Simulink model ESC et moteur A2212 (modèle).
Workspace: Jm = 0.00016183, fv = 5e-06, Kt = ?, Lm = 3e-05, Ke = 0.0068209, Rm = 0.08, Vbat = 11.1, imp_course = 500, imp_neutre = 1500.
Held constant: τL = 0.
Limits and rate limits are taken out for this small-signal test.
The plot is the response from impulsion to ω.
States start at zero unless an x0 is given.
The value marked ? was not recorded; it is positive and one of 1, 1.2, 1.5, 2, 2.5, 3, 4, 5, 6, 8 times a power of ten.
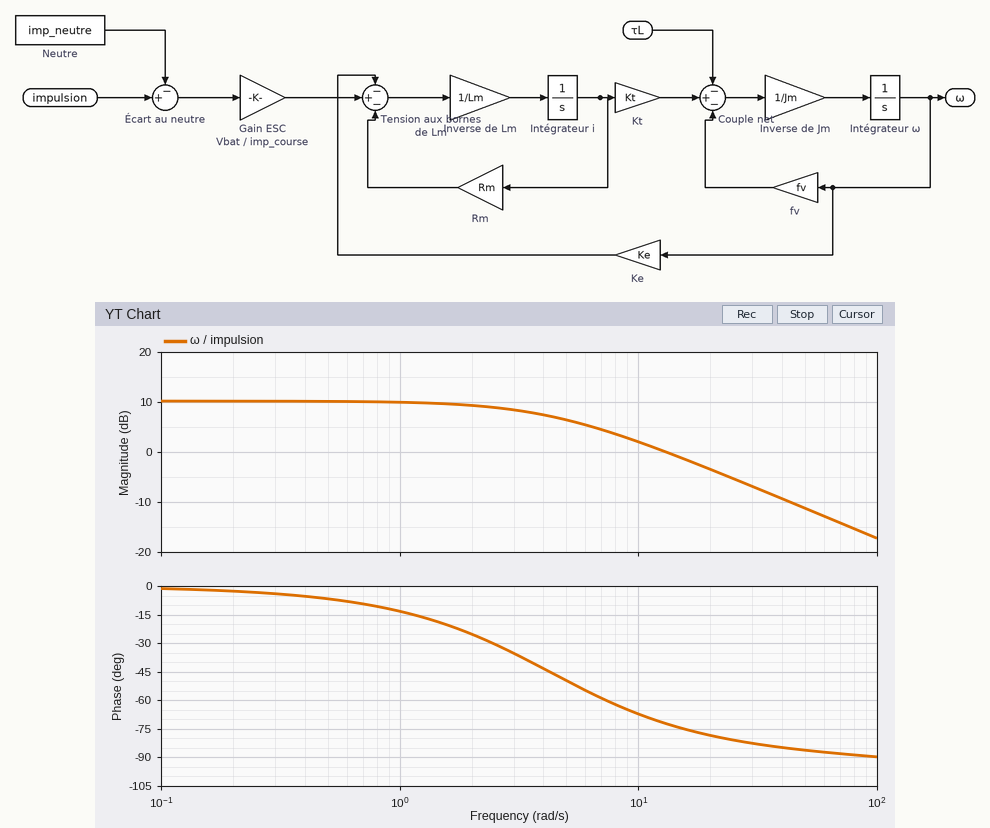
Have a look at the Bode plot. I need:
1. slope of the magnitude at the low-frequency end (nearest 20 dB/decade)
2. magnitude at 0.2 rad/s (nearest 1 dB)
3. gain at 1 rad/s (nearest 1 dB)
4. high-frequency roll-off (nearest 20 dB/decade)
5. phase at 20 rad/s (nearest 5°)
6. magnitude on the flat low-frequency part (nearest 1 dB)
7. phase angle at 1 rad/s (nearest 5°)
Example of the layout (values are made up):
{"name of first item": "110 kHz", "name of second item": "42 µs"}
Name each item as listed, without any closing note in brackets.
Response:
{"slope of the magnitude at the low-frequency end": "0 dB/decade", "magnitude at 0.2 rad/s": "10 dB", "gain at 1 rad/s": "10 dB", "high-frequency roll-off": "-20 dB/decade", "phase at 20 rad/s": "-80°", "magnitude on the flat low-frequency part": "10 dB", "phase angle at 1 rad/s": "-15°"}
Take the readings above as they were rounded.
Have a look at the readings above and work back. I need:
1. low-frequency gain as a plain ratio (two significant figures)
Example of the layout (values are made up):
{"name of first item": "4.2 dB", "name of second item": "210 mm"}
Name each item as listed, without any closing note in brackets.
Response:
{"low-frequency gain as a plain ratio": "3.2"}
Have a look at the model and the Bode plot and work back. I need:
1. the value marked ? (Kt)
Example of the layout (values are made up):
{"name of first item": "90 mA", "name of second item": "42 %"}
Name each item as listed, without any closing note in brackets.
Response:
{"the value marked ?": "0.008"}
